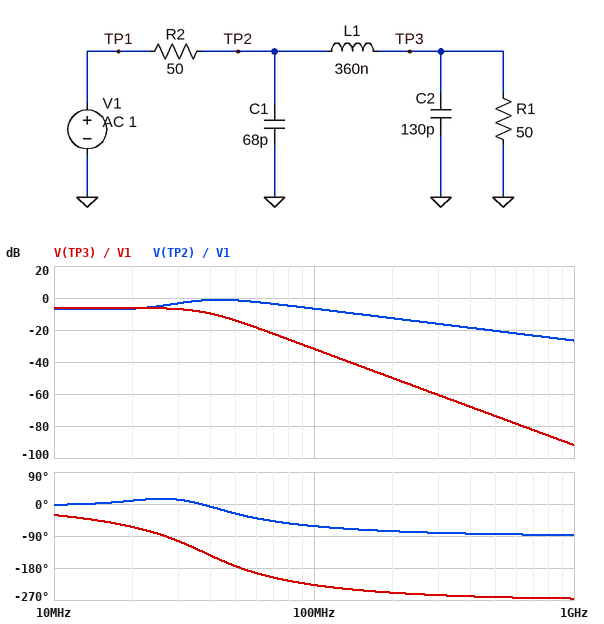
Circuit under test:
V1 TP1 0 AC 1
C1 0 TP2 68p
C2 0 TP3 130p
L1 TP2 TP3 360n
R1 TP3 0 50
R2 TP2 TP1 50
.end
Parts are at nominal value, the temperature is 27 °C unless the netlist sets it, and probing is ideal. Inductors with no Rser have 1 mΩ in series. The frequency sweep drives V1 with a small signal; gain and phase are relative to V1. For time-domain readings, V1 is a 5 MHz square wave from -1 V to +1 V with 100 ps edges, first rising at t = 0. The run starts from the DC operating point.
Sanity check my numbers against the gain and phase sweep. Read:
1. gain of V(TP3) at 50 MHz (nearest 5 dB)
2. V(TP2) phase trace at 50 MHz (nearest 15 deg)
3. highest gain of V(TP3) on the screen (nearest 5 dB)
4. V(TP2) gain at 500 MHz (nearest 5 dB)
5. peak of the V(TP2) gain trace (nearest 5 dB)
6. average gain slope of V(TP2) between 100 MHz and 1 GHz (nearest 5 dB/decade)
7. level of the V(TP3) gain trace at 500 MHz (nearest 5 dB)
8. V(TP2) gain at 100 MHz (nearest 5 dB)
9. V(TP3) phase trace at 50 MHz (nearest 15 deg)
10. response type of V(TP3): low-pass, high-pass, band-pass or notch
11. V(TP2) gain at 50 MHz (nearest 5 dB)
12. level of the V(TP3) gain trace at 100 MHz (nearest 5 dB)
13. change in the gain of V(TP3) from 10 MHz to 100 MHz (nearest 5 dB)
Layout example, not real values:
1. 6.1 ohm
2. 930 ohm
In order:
1. -15 dB
2. -30 deg
3. -5 dB
4. -20 dB
5. 0 dB
6. -20 dB/decade
7. -75 dB
8. -5 dB
9. -180 deg
10. low-pass
11. 0 dB
12. -30 dB
13. -25 dB
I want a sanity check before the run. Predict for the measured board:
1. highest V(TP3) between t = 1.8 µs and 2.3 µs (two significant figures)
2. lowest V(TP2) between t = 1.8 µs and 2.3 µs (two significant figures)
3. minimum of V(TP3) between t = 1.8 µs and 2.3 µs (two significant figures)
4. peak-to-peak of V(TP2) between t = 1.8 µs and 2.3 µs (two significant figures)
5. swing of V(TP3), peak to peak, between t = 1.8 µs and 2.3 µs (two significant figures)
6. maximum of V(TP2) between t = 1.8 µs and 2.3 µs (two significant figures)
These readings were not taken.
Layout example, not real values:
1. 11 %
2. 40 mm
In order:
1. 580 mV
2. -820 mV
3. -580 mV
4. 1.6 V
5. 1.2 V
6. 820 mV
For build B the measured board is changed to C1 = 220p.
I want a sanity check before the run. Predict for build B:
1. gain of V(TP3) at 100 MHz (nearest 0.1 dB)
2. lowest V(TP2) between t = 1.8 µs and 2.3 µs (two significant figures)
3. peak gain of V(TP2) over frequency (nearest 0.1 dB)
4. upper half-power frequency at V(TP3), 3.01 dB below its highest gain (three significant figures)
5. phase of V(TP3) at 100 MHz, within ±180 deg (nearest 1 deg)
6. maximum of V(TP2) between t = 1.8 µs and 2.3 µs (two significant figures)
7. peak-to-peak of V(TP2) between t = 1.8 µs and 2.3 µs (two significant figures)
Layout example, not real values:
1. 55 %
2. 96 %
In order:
1. -41.7 dB
2. -520 mV
3. -5.2 dB
4. 30.4 MHz
5. 113 deg
6. 520 mV
7. 1.0 V
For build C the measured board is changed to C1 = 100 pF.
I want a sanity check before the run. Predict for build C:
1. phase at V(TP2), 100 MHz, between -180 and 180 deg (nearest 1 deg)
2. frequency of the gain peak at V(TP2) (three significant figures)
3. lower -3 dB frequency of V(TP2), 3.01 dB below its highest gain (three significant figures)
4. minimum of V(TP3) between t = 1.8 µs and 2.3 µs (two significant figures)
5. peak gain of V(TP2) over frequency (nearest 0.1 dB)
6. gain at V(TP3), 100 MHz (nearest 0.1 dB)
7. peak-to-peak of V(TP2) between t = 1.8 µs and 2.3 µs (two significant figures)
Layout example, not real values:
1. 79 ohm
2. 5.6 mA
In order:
1. -71 deg
2. 37.6 MHz
3. 25.1 MHz
4. -600 mV
5. -2.0 dB
6. -34.9 dB
7. 1.4 V
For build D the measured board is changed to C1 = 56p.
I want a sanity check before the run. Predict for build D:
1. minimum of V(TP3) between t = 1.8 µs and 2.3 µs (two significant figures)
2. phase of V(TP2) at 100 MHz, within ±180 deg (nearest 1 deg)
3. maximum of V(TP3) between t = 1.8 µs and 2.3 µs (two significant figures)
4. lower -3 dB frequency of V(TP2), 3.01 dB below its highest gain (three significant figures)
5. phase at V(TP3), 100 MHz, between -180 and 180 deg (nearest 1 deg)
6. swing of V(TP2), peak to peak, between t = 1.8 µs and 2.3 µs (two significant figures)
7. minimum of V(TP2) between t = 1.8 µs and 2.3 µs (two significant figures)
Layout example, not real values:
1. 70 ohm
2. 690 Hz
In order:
1. -570 mV
2. -57 deg
3. 570 mV
4. 29.1 MHz
5. 138 deg
6. 1.7 V
7. -870 mV
